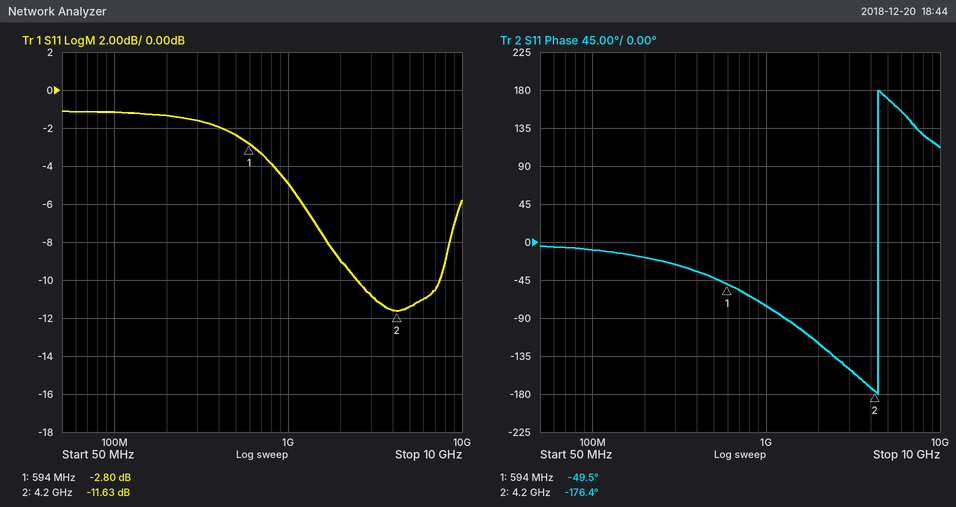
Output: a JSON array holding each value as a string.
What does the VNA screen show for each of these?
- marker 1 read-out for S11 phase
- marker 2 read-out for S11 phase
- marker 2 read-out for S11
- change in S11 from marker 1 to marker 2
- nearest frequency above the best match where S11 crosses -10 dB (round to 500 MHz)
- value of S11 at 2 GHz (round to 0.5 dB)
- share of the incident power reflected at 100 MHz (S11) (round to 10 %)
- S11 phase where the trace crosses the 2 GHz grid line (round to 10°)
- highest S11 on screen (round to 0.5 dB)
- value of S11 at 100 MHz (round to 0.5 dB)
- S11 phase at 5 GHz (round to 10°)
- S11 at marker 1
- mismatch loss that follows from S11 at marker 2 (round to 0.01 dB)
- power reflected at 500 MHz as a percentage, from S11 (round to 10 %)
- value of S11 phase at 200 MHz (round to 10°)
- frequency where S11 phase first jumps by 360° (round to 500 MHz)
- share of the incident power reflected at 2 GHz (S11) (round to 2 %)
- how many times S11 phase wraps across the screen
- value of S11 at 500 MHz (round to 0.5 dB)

["-49.5°", "-176.4°", "-11.63 dB", "-8.83 dB", "7.5 GHz", "-9.0 dB", "80 %", "-120°", "-1.0 dB", "-1.0 dB", "170°", "-2.80 dB", "0.31 dB", "60 %", "-20°", "4.5 GHz", "12 %", "1", "-2.5 dB"]
